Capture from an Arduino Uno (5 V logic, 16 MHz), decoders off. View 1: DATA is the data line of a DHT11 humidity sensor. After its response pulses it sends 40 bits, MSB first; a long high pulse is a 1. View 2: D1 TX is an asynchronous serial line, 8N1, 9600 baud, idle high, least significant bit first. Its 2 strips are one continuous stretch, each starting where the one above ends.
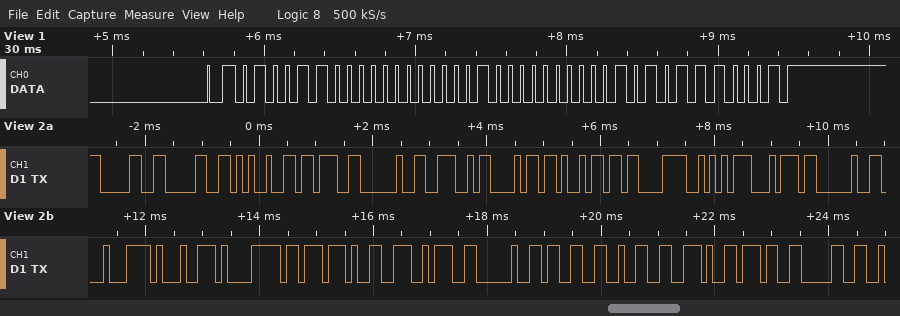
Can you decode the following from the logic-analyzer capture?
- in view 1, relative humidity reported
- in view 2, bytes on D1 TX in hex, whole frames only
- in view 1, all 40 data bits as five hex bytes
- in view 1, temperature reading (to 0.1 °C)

76 %
0x30 0x30 0x25 0x3B 0x20 0x4E 0x68 0x69 0xC3 0xAA 0x74 0x20 0xC4 0x91 0xE1 0xBB 0x99 0x3A 0x20 0x33 0x32 0x2E 0x37 0x30
4C 00 20 05 71
32.5 °C
